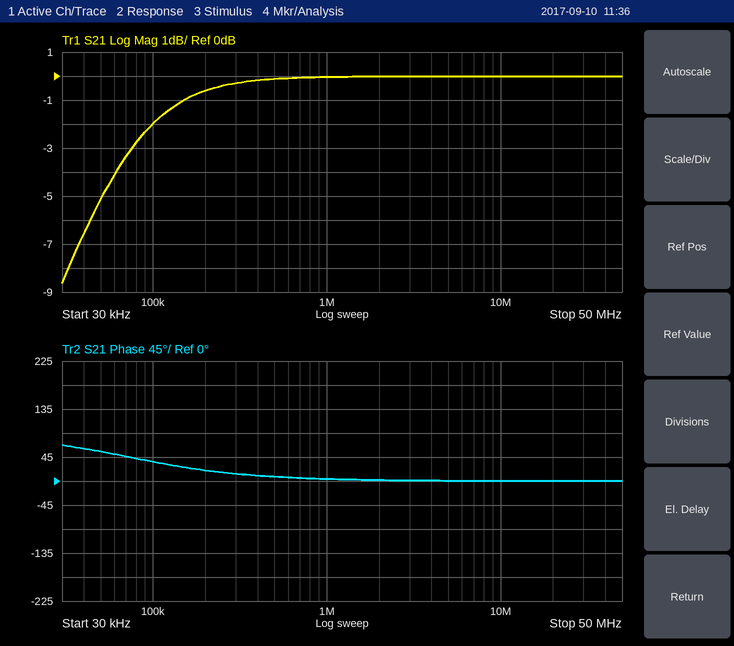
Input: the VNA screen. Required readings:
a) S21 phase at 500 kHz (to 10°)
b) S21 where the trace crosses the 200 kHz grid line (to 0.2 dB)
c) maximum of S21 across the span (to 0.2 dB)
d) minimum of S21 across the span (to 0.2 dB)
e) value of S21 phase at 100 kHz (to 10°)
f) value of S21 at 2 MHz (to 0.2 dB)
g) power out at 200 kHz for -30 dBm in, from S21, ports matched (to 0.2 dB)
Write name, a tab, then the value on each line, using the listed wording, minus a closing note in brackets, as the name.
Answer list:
S21 phase at 500 kHz	10°
S21 where the trace crosses the 200 kHz grid line	-0.6 dB
maximum of S21 across the span	0.0 dB
minimum of S21 across the span	-8.6 dB
value of S21 phase at 100 kHz	40°
value of S21 at 2 MHz	0.0 dB
power out at 200 kHz for -30 dBm in, from S21, ports matched	-30.6 dBm
